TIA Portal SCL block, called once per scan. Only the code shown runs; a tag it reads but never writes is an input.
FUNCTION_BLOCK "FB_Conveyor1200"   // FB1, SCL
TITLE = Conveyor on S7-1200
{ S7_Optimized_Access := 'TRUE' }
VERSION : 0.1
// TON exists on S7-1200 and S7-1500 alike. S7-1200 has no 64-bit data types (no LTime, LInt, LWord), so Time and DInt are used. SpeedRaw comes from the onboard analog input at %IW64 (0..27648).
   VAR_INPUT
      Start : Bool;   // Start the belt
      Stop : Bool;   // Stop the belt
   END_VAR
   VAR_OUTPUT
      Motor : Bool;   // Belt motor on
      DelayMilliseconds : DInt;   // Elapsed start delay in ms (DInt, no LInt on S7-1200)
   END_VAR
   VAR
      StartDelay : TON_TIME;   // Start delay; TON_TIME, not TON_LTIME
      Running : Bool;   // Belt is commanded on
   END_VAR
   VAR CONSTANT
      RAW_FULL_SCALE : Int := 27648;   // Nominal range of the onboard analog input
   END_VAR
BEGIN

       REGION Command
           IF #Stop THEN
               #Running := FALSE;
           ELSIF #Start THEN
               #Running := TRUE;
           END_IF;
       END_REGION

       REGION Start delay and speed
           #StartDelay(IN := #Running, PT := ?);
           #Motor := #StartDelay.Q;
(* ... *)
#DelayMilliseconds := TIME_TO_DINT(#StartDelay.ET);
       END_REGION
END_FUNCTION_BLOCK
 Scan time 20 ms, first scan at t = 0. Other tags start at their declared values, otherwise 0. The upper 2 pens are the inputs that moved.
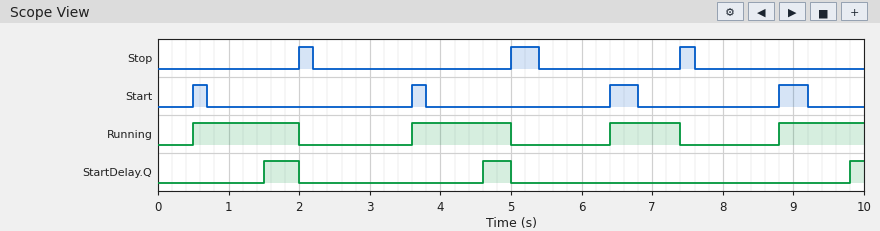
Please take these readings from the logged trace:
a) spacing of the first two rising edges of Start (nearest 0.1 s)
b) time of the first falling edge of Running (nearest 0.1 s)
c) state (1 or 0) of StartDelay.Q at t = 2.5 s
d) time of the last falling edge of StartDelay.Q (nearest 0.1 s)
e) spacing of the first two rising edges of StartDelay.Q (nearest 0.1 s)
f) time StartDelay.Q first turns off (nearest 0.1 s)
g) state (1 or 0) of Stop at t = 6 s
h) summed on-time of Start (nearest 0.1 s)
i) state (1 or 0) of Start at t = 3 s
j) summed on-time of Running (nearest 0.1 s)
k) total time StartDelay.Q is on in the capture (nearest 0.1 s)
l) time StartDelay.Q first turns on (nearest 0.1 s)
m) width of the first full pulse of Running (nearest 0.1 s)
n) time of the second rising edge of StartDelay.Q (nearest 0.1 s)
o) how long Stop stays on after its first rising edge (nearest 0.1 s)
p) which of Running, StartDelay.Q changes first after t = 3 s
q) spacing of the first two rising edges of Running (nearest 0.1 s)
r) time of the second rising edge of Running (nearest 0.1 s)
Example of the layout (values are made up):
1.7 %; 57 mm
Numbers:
3.1 s; 2.0 s; 0; 5.0 s; 3.1 s; 2.0 s; 0; 1.2 s; 0; 5.1 s; 1.1 s; 1.5 s; 1.5 s; 4.6 s; 0.2 s; Running; 3.1 s; 3.6 s
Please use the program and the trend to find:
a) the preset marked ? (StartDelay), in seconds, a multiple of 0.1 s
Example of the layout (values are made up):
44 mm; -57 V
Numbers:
1.0 s
